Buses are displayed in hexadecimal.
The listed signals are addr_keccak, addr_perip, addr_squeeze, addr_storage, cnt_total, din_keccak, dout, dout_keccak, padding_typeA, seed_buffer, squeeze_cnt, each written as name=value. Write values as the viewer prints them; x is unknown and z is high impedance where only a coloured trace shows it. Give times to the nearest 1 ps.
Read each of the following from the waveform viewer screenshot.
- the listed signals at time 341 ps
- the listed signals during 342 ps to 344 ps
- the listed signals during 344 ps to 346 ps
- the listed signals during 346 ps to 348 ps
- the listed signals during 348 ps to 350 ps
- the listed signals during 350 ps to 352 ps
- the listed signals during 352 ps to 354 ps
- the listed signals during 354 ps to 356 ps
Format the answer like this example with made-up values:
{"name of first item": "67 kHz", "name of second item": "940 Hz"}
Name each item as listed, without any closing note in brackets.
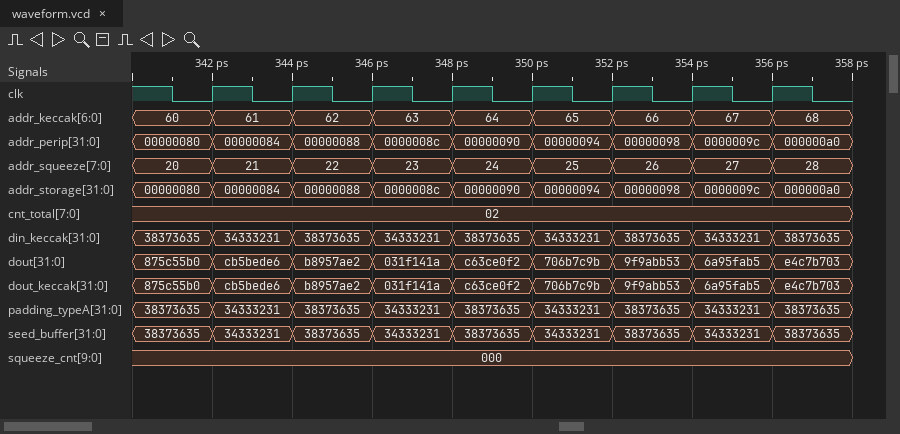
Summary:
{"the listed signals at time 341 ps": "addr_keccak=60, addr_perip=00000080, addr_squeeze=20, addr_storage=00000080, cnt_total=02, din_keccak=38373635, dout=875c55b0, dout_keccak=875c55b0, padding_typeA=38373635, seed_buffer=38373635, squeeze_cnt=000", "the listed signals during 342 ps to 344 ps": "addr_keccak=61, addr_perip=00000084, addr_squeeze=21, addr_storage=00000084, cnt_total=02, din_keccak=34333231, dout=cb5bede6, dout_keccak=cb5bede6, padding_typeA=34333231, seed_buffer=34333231, squeeze_cnt=000", "the listed signals during 344 ps to 346 ps": "addr_keccak=62, addr_perip=00000088, addr_squeeze=22, addr_storage=00000088, cnt_total=02, din_keccak=38373635, dout=b8957ae2, dout_keccak=b8957ae2, padding_typeA=38373635, seed_buffer=38373635, squeeze_cnt=000", "the listed signals during 346 ps to 348 ps": "addr_keccak=63, addr_perip=0000008c, addr_squeeze=23, addr_storage=0000008c, cnt_total=02, din_keccak=34333231, dout=031f141a, dout_keccak=031f141a, padding_typeA=34333231, seed_buffer=34333231, squeeze_cnt=000", "the listed signals during 348 ps to 350 ps": "addr_keccak=64, addr_perip=00000090, addr_squeeze=24, addr_storage=00000090, cnt_total=02, din_keccak=38373635, dout=c63ce0f2, dout_keccak=c63ce0f2, padding_typeA=38373635, seed_buffer=38373635, squeeze_cnt=000", "the listed signals during 350 ps to 352 ps": "addr_keccak=65, addr_perip=00000094, addr_squeeze=25, addr_storage=00000094, cnt_total=02, din_keccak=34333231, dout=706b7c9b, dout_keccak=706b7c9b, padding_typeA=34333231, seed_buffer=34333231, squeeze_cnt=000", "the listed signals during 352 ps to 354 ps": "addr_keccak=66, addr_perip=00000098, addr_squeeze=26, addr_storage=00000098, cnt_total=02, din_keccak=38373635, dout=9f9abb53, dout_keccak=9f9abb53, padding_typeA=38373635, seed_buffer=38373635, squeeze_cnt=000", "the listed signals during 354 ps to 356 ps": "addr_keccak=67, addr_perip=0000009c, addr_squeeze=27, addr_storage=0000009c, cnt_total=02, din_keccak=34333231, dout=6a95fab5, dout_keccak=6a95fab5, padding_typeA=34333231, seed_buffer=34333231, squeeze_cnt=000"}
